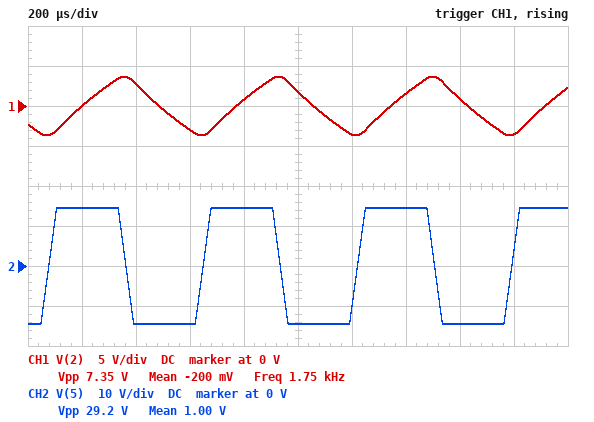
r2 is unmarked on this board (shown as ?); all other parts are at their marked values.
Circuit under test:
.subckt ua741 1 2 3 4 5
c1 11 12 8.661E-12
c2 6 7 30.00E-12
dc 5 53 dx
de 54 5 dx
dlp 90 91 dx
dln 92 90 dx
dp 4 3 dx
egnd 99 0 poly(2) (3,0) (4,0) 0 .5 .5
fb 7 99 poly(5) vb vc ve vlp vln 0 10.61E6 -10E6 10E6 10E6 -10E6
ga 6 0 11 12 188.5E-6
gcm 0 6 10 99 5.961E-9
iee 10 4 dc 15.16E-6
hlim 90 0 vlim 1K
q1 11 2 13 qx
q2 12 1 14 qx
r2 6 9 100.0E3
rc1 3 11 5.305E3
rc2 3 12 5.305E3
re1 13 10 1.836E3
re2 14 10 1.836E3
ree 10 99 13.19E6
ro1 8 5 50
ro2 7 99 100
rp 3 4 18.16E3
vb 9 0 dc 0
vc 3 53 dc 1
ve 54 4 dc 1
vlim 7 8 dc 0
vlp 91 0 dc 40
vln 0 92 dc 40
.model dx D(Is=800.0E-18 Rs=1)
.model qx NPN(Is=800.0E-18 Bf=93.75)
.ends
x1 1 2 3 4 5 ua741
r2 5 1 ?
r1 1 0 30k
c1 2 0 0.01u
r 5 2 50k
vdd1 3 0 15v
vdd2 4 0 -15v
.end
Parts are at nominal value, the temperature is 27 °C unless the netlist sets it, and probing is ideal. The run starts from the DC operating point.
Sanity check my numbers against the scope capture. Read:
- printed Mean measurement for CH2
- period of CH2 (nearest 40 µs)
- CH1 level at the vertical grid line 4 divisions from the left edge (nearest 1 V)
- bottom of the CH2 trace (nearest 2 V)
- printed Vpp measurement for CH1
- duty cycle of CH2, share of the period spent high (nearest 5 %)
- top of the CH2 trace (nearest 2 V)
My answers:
1.00 V
560 µs
1 V
-14 V
7.35 V
50 %
14 V
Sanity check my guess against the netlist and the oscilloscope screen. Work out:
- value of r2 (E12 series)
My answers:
100 kΩ
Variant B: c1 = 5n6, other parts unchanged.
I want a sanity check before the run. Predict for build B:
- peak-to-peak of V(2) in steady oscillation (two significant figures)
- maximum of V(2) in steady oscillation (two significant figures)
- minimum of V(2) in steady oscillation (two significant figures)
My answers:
7.8 V
3.9 V
-3.9 V
